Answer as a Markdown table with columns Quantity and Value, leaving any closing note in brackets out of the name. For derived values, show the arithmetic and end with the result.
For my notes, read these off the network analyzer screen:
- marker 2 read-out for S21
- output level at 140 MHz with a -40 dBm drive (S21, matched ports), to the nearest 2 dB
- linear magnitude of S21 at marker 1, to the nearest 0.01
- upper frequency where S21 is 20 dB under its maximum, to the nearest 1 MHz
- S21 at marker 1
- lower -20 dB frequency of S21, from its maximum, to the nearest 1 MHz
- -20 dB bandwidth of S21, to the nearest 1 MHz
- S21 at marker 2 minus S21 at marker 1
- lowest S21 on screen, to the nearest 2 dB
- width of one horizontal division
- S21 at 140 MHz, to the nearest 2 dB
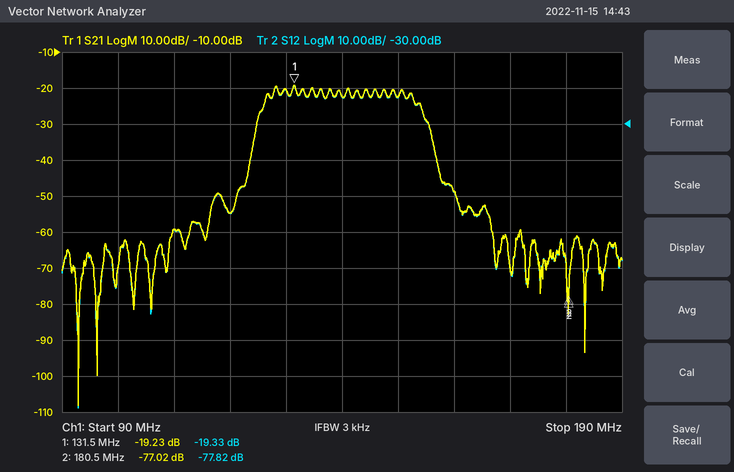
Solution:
| Quantity | Value |
|---|---|
| marker 2 read-out for S21 | -77.02 dB |
| output level at 140 MHz with a -40 dBm drive (S21, matched ports), to the nearest 2 dB | -40 dBm + (-22 dB) = -62 dBm |
| linear magnitude of S21 at marker 1, to the nearest 0.01 | 10^(-19.23/20) ≈ 0.11 |
| upper frequency where S21 is 20 dB under its maximum, to the nearest 1 MHz | 157 MHz |
| S21 at marker 1 | -19.23 dB |
| lower -20 dB frequency of S21, from its maximum, to the nearest 1 MHz | 124 MHz |
| -20 dB bandwidth of S21, to the nearest 1 MHz | 157 MHz − 124 MHz = 33 MHz |
| S21 at marker 2 minus S21 at marker 1 | -77.02 − (-19.23) = -57.79 dB |
| lowest S21 on screen, to the nearest 2 dB | -108 dB |
| width of one horizontal division | 10 MHz |
| S21 at 140 MHz, to the nearest 2 dB | -22 dB |
